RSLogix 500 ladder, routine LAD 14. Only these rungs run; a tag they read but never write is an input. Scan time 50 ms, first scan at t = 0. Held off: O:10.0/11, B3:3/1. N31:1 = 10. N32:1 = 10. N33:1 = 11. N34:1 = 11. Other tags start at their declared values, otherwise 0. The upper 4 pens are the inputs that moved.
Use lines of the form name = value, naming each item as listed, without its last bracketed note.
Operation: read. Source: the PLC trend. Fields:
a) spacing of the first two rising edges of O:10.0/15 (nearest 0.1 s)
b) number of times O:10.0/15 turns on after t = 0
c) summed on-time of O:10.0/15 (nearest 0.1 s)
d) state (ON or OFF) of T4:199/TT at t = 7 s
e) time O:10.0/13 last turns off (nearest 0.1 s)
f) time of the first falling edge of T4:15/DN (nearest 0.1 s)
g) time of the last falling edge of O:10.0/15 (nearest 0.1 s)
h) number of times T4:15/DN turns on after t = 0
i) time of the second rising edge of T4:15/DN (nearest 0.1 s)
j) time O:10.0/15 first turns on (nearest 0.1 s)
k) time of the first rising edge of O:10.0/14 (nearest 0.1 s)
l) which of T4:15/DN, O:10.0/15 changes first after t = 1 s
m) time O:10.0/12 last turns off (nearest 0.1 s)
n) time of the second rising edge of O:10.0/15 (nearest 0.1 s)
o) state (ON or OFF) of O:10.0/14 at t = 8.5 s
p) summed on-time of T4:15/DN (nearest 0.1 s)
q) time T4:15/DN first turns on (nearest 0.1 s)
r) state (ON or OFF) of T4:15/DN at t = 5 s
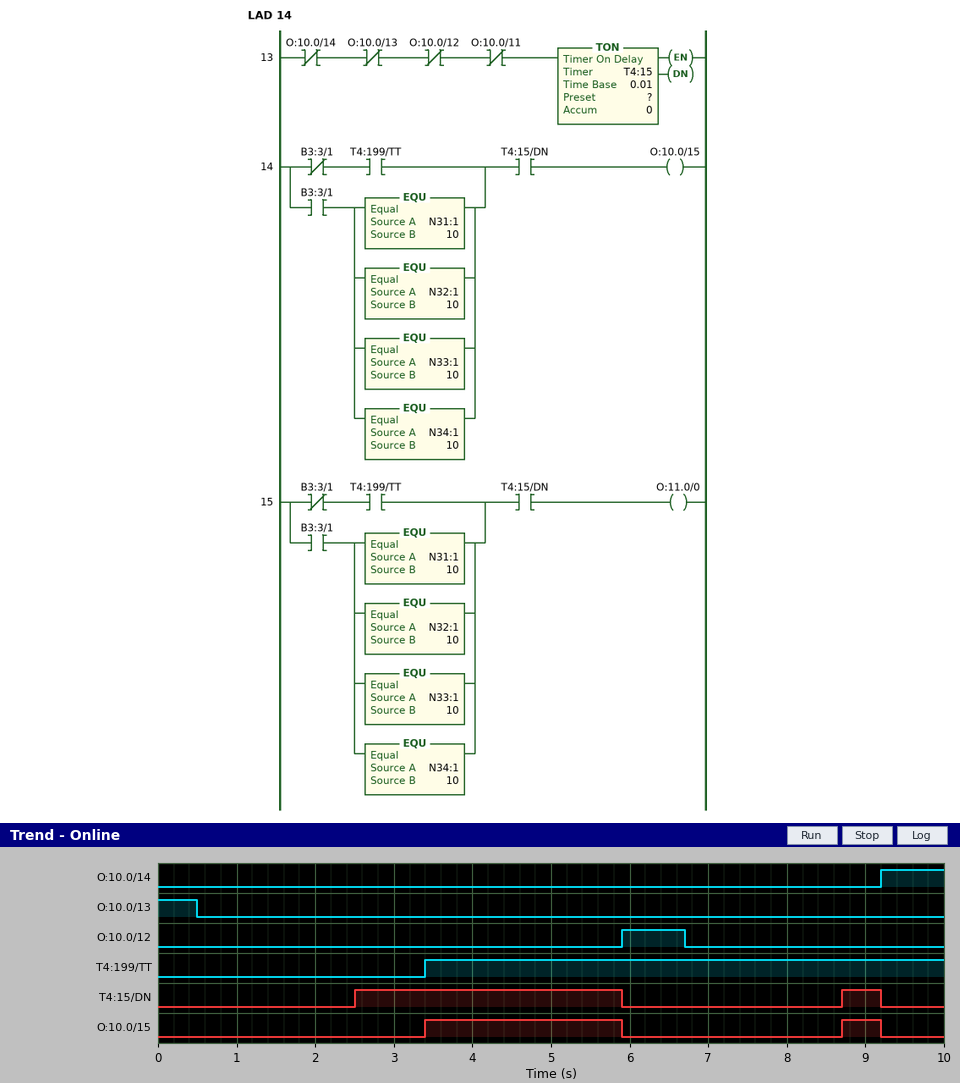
spacing of the first two rising edges of O:10.0/15 = 5.3 s
number of times O:10.0/15 turns on after t = 0 = 2
summed on-time of O:10.0/15 = 3.0 s
state (ON or OFF) of T4:199/TT at t = 7 s = ON
time O:10.0/13 last turns off = 0.5 s
time of the first falling edge of T4:15/DN = 5.9 s
time of the last falling edge of O:10.0/15 = 9.2 s
number of times T4:15/DN turns on after t = 0 = 2
time of the second rising edge of T4:15/DN = 8.7 s
time O:10.0/15 first turns on = 3.4 s
time of the first rising edge of O:10.0/14 = 9.2 s
which of T4:15/DN, O:10.0/15 changes first after t = 1 s = T4:15/DN
time O:10.0/12 last turns off = 6.7 s
time of the second rising edge of O:10.0/15 = 8.7 s
state (ON or OFF) of O:10.0/14 at t = 8.5 s = OFF
summed on-time of T4:15/DN = 3.9 s
time T4:15/DN first turns on = 2.5 s
state (ON or OFF) of T4:15/DN at t = 5 s = ON
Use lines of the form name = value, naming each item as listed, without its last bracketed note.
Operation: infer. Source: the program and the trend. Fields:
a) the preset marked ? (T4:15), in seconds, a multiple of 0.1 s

the preset marked ? (T4:15), in seconds, a multiple of 0.1 s = 2.0 s
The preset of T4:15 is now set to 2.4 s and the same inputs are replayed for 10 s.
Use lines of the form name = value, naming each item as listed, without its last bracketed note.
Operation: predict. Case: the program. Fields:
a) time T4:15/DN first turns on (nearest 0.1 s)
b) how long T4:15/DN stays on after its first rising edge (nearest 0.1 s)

time T4:15/DN first turns on = 2.9 s
how long T4:15/DN stays on after its first rising edge = 3.0 s
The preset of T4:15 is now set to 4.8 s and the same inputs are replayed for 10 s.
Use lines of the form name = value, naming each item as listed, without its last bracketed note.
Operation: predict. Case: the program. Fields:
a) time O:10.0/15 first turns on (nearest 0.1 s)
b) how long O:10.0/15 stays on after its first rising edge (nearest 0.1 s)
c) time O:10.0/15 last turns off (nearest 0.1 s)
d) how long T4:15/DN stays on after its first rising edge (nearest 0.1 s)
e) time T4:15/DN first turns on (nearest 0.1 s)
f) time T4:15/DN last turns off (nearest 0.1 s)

time O:10.0/15 first turns on = 5.3 s
how long O:10.0/15 stays on after its first rising edge = 0.6 s
time O:10.0/15 last turns off = 5.9 s
how long T4:15/DN stays on after its first rising edge = 0.6 s
time T4:15/DN first turns on = 5.3 s
time T4:15/DN last turns off = 5.9 s
